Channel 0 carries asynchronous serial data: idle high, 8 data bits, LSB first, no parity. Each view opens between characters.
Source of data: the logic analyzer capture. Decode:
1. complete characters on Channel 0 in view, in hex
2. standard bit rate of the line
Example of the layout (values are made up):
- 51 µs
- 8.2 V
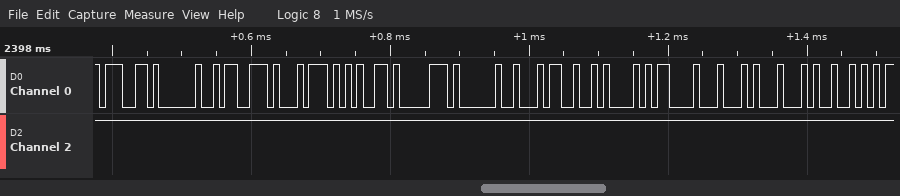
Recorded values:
- 67, 20, 73, 74, 65, 70, 20, 34, 0A, 0D, 44, 44, 52
- 115200 baud
